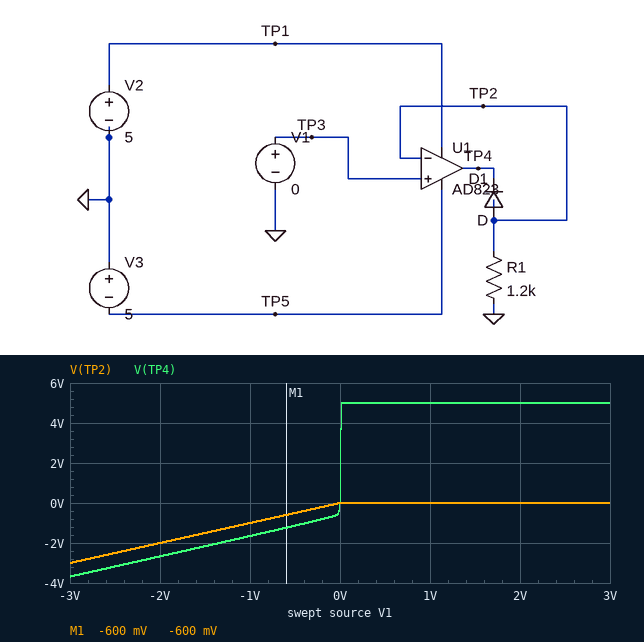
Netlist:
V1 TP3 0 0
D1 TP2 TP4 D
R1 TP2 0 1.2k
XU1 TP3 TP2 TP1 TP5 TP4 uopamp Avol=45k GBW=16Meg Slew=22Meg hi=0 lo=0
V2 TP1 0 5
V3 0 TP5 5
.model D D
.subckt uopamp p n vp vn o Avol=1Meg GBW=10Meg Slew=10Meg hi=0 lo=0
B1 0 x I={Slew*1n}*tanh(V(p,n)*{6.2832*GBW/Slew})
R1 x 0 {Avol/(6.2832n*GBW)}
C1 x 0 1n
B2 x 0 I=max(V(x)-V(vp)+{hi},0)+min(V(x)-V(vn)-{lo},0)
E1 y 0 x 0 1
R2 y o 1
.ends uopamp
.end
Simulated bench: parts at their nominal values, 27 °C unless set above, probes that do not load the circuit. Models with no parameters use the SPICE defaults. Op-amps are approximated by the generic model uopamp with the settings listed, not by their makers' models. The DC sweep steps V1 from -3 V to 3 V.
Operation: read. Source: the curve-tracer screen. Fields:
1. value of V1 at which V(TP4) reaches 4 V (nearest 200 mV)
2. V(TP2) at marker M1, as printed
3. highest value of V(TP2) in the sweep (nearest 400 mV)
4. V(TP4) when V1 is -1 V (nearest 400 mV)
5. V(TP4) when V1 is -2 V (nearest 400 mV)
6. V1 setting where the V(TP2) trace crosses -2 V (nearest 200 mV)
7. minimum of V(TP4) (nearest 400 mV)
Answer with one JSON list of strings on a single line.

["0 V", "-600 mV", "0 V", "-1.6 V", "-2.8 V", "-2.0 V", "-3.6 V"]
